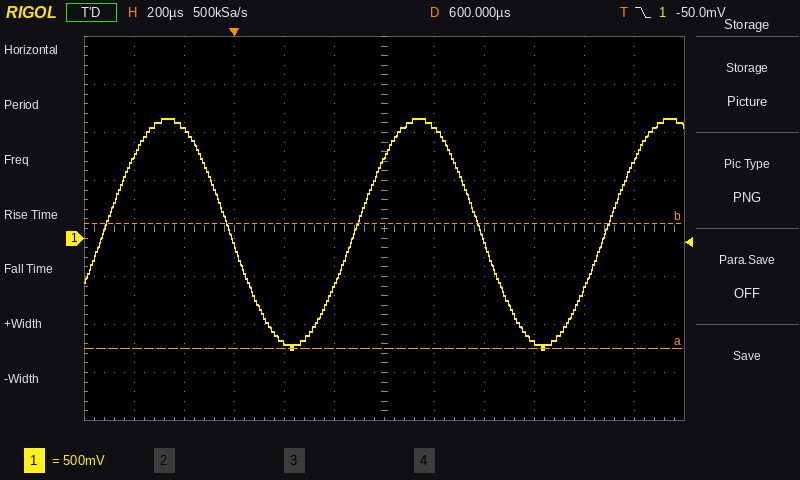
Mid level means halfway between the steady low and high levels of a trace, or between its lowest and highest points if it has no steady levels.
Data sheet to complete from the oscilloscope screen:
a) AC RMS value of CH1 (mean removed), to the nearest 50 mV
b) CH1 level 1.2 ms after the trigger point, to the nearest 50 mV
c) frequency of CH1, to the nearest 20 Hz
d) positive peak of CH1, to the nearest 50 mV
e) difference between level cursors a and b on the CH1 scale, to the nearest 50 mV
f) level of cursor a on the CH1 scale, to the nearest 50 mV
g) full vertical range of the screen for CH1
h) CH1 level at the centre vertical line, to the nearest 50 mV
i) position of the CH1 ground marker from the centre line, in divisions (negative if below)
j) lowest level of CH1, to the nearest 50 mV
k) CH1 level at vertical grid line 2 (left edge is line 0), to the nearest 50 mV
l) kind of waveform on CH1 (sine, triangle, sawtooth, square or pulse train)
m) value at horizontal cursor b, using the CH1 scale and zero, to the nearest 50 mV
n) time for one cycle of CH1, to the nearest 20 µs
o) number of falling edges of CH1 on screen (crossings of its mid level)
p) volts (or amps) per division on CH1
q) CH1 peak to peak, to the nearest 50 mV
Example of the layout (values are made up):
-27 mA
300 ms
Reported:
850 mV
-1.10 V
1.00 kHz
1.25 V
1.30 V
-1.15 V
4 V
850 mV
-0.2 div
-1.15 V
1.15 V
sine
150 mV
1.00 ms
2
500 mV
2.40 V
